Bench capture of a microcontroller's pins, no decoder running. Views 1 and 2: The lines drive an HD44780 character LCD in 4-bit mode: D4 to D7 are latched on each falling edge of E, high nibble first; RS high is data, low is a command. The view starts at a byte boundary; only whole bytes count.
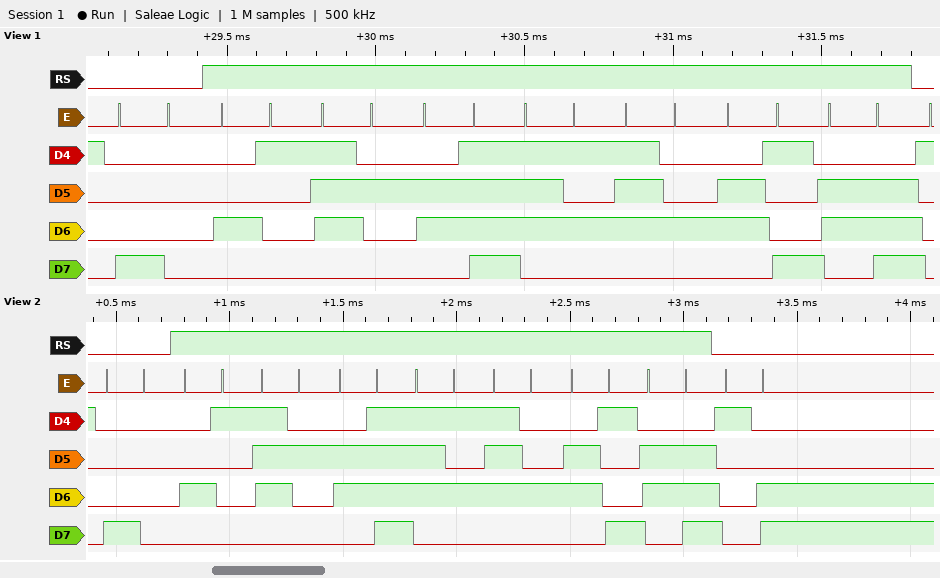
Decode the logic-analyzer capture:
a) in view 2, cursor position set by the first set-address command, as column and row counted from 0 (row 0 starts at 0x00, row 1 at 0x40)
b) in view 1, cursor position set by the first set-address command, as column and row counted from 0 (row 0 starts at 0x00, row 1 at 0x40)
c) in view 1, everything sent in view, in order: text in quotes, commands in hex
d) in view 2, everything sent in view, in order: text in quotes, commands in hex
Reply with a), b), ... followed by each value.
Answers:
a) column 0, row 0
b) column 0, row 0
c) 0x80 "Aroutin"
d) 0x80 "Aroutin" 0x1C
